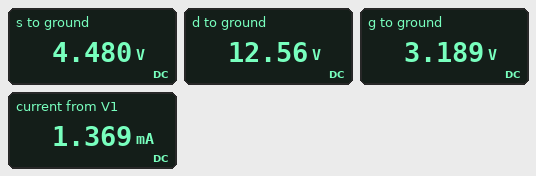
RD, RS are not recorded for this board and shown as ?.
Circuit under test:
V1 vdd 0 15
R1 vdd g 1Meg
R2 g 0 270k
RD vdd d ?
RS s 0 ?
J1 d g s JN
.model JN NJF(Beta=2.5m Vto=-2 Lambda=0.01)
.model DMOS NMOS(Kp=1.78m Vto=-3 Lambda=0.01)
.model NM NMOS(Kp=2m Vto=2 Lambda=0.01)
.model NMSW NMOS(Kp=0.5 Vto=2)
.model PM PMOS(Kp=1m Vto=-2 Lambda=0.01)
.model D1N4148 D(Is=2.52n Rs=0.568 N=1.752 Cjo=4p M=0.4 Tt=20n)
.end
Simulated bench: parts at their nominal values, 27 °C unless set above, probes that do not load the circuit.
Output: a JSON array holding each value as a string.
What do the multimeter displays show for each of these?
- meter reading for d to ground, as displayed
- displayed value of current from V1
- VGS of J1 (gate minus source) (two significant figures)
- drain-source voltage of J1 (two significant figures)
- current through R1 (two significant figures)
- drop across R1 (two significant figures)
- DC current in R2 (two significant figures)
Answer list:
["12.56 V", "1.369 mA", "-1.3 V", "8.1 V", "12 µA", "12 V", "12 µA"]
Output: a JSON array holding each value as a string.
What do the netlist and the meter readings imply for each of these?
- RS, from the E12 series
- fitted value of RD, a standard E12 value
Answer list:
["3.3 kΩ", "1.8 kΩ"]
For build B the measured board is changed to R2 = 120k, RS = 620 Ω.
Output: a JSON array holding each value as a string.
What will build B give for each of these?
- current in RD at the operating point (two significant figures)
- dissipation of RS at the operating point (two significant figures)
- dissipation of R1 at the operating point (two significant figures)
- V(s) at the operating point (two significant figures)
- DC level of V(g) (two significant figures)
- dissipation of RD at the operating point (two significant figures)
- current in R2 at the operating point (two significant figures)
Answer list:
["3.9 mA", "9.3 mW", "180 µW", "2.4 V", "1.6 V", "27 mW", "13 µA"]
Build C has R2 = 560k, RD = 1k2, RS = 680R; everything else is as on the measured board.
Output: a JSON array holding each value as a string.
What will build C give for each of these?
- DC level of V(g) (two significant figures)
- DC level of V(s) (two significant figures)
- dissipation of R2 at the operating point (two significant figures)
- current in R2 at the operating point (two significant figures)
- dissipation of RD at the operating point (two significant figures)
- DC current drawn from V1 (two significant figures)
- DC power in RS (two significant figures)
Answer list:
["5.4 V", "5.1 V", "52 µW", "9.6 µA", "68 mW", "7.6 mA", "39 mW"]
